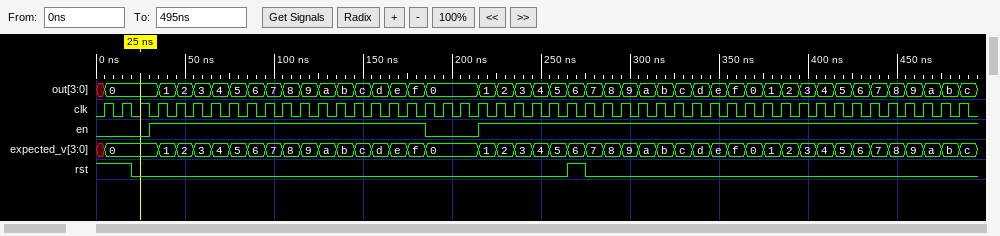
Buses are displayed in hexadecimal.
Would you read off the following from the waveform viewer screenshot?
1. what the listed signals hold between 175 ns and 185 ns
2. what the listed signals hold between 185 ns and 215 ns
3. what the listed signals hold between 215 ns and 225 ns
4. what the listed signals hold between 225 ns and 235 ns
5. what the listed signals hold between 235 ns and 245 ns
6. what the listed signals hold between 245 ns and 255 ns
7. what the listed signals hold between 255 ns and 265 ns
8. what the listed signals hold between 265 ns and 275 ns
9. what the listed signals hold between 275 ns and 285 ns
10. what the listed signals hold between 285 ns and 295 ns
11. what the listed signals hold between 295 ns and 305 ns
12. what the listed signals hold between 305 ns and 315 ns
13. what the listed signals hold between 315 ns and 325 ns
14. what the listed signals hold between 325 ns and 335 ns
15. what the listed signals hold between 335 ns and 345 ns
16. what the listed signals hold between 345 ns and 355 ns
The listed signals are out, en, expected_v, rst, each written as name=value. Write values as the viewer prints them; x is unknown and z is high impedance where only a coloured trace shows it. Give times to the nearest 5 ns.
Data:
out=f, en=1, expected_v=f, rst=0
out=0, en=0, expected_v=0, rst=0
out=1, en=1, expected_v=1, rst=0
out=2, en=1, expected_v=2, rst=0
out=3, en=1, expected_v=3, rst=0
out=4, en=1, expected_v=4, rst=0
out=5, en=1, expected_v=5, rst=0
out=6, en=1, expected_v=6, rst=1
out=7, en=1, expected_v=7, rst=0
out=8, en=1, expected_v=8, rst=0
out=9, en=1, expected_v=9, rst=0
out=a, en=1, expected_v=a, rst=0
out=b, en=1, expected_v=b, rst=0
out=c, en=1, expected_v=c, rst=0
out=d, en=1, expected_v=d, rst=0
out=e, en=1, expected_v=e, rst=0
